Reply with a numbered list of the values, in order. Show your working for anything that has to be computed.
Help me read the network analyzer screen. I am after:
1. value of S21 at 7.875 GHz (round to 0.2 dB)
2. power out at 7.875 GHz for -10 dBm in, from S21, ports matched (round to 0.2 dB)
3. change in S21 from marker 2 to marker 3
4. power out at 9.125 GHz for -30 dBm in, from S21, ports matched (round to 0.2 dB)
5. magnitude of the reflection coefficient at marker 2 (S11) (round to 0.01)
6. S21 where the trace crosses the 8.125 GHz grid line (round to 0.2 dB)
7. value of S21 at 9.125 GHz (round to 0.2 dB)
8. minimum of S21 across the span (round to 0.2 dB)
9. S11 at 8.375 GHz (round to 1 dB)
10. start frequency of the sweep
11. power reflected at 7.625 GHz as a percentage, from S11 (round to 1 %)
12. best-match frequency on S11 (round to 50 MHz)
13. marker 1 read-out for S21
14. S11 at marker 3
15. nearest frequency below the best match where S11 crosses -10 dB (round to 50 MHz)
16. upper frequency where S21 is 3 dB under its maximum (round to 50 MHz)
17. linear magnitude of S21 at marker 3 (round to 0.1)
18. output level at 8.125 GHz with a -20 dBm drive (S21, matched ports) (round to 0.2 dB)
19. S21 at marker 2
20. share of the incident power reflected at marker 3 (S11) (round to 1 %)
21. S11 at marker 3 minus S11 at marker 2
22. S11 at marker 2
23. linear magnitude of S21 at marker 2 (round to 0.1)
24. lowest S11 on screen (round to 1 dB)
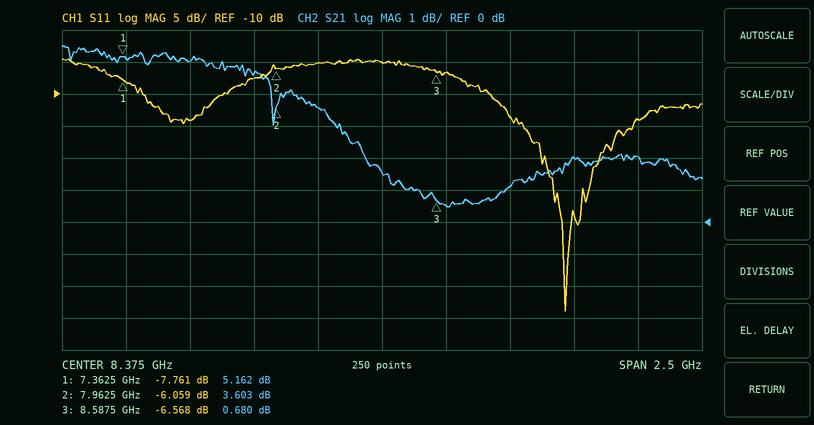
1. 4.6 dB
2. -10 dBm + (4.6 dB) = -5.4 dBm
3. 0.68 − (3.603) = -2.923 dB
4. -30 dBm + (2.0 dB) = -28.0 dBm
5. 10^(-6.059/20) ≈ 0.50
6. 3.6 dB
7. 2.0 dB
8. 0.4 dB
9. -5 dB
10. 7.125 GHz
11. 10^(-14/10) ≈ 4 %
12. 9.10 GHz
13. 5.162 dB
14. -6.568 dB
15. 8.80 GHz
16. 8.25 GHz
17. 10^(0.68/20) ≈ 1.1
18. -20 dBm + (3.6 dB) = -16.4 dBm
19. 3.603 dB
20. 10^(-6.568/10) ≈ 22 %
21. -6.568 − (-6.059) = -0.509 dB
22. -6.059 dB
23. 10^(3.603/20) ≈ 1.5
24. -44 dB
